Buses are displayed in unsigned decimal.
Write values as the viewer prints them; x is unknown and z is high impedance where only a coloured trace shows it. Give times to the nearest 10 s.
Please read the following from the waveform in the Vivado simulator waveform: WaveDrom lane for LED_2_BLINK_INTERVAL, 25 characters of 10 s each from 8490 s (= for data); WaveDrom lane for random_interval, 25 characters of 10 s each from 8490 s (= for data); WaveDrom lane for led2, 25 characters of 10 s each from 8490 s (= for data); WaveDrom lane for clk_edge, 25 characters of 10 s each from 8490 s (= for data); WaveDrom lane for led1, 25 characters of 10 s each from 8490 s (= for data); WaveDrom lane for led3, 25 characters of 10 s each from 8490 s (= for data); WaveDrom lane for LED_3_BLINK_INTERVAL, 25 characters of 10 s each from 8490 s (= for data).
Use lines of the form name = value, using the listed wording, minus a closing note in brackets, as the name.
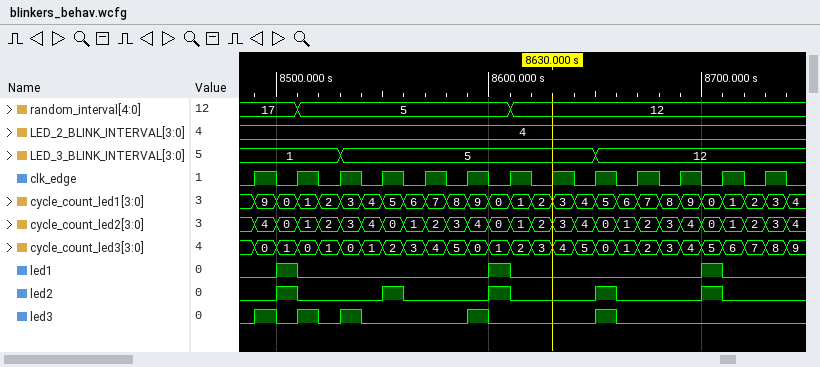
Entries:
WaveDrom lane for LED_2_BLINK_INTERVAL, 25 characters of 10 s each from 8490 s = {name: 'LED_2_BLINK_INTERVAL', wave: '=........................', data: '4'}
WaveDrom lane for random_interval, 25 characters of 10 s each from 8490 s = {name: 'random_interval', wave: '=.=.........=............', data: '17 5 12'}
WaveDrom lane for led2, 25 characters of 10 s each from 8490 s = {name: 'led2', wave: '010...10...10...10...10..'}
WaveDrom lane for clk_edge, 25 characters of 10 s each from 8490 s = {name: 'clk_edge', wave: '1010101010101010101010101'}
WaveDrom lane for led1, 25 characters of 10 s each from 8490 s = {name: 'led1', wave: '010........10........10..'}
WaveDrom lane for led3, 25 characters of 10 s each from 8490 s = {name: 'led3', wave: '101010....10....10.......'}
WaveDrom lane for LED_3_BLINK_INTERVAL, 25 characters of 10 s each from 8490 s = {name: 'LED_3_BLINK_INTERVAL', wave: '=...=...........=........', data: '1 5 12'}
